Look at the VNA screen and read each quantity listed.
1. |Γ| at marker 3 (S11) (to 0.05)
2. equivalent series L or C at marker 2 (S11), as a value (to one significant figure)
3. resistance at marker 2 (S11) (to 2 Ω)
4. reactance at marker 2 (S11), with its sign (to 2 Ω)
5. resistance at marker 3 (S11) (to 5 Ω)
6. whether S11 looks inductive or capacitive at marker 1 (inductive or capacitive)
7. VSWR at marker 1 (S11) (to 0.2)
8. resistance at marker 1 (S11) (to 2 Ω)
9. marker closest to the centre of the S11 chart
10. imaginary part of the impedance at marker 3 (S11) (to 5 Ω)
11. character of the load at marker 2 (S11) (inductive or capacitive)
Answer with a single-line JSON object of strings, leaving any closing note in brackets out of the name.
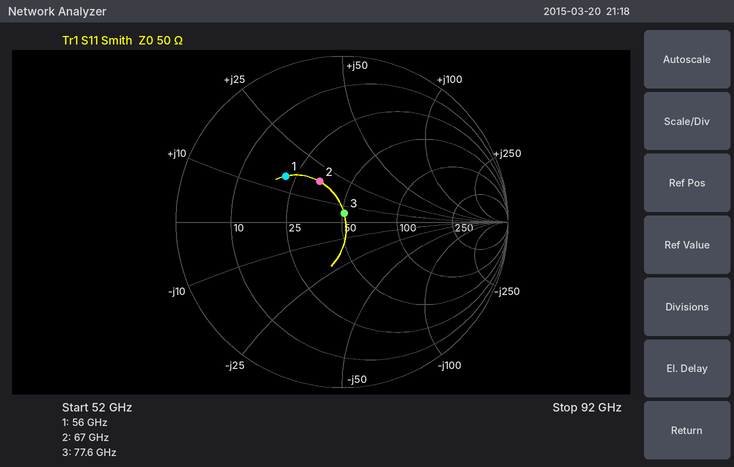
{"|Γ| at marker 3 (S11)": "0.05", "equivalent series L or C at marker 2 (S11), as a value": "40 pH", "resistance at marker 2 (S11)": "34 Ω", "reactance at marker 2 (S11), with its sign": "+18 Ω", "resistance at marker 3 (S11)": "50 Ω", "whether S11 looks inductive or capacitive at marker 1": "inductive", "VSWR at marker 1 (S11)": "2.6", "resistance at marker 1 (S11)": "22 Ω", "marker closest to the centre of the S11 chart": "marker 3", "imaginary part of the impedance at marker 3 (S11)": "+5 Ω", "character of the load at marker 2 (S11)": "inductive"}
